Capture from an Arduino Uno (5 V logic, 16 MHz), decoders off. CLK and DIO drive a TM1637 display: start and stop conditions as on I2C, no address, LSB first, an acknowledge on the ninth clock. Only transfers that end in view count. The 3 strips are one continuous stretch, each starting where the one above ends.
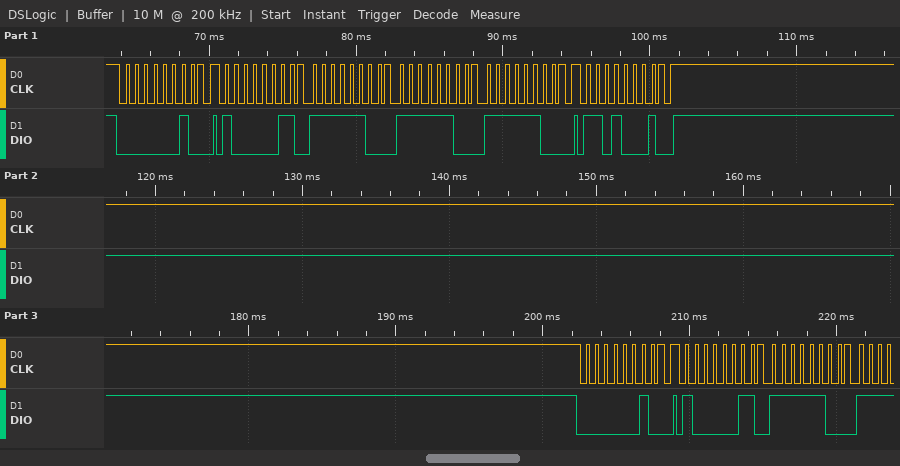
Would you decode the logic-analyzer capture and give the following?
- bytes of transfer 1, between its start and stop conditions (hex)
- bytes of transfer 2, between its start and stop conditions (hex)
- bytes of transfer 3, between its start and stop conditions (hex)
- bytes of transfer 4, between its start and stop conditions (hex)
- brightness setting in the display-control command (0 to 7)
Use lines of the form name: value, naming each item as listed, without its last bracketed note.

bytes of transfer 1, between its start and stop conditions: 40
bytes of transfer 2, between its start and stop conditions: C1 3F 3F 3F
bytes of transfer 3, between its start and stop conditions: 8B
bytes of transfer 4, between its start and stop conditions: 40
brightness setting in the display-control command: 3
